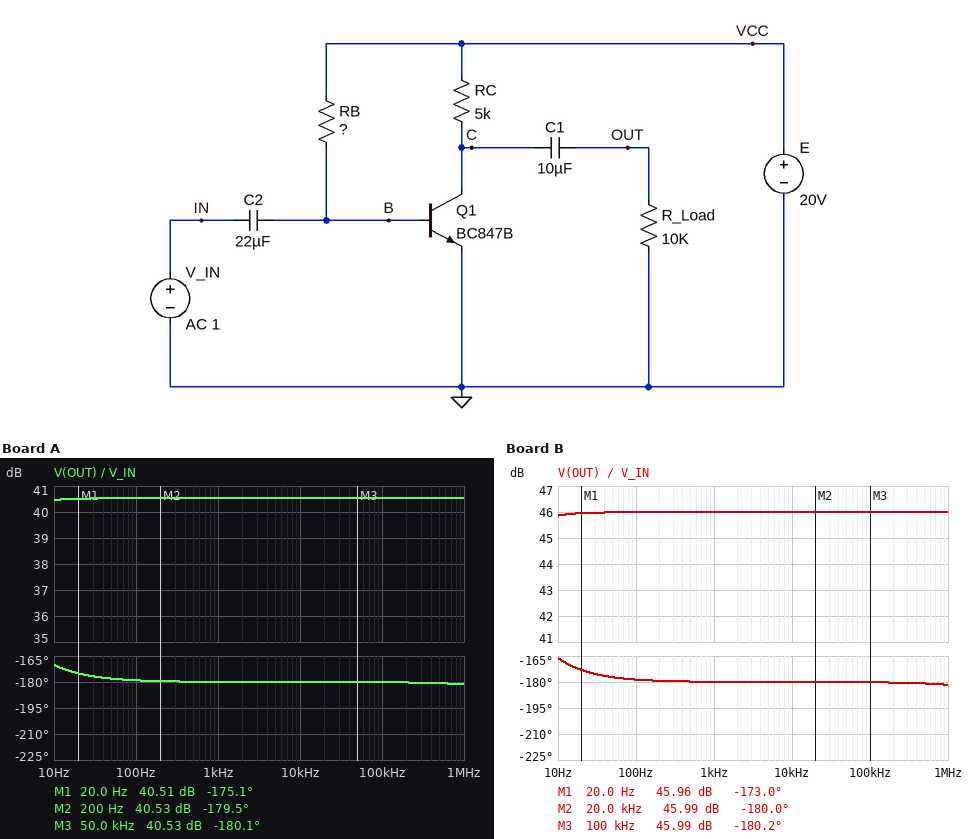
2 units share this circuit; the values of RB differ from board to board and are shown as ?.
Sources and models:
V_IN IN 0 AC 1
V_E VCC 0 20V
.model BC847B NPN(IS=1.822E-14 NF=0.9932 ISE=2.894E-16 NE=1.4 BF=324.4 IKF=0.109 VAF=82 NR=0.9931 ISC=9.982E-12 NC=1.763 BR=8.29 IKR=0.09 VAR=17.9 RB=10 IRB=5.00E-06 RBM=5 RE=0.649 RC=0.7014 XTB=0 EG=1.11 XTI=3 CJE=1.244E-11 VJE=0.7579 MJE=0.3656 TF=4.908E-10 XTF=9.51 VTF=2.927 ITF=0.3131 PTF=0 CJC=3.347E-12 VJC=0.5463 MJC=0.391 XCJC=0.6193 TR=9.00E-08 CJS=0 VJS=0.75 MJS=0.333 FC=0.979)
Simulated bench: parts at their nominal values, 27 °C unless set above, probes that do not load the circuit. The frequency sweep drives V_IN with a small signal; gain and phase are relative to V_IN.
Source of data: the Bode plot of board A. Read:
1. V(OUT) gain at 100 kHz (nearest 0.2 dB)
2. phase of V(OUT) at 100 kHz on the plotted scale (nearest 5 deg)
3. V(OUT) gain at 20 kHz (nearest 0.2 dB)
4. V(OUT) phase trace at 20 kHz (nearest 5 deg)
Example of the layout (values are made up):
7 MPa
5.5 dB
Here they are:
40.6 dB
-180 deg
40.6 dB
-180 deg
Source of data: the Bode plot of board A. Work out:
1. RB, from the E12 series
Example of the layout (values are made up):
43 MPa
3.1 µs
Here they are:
8.2 MΩ
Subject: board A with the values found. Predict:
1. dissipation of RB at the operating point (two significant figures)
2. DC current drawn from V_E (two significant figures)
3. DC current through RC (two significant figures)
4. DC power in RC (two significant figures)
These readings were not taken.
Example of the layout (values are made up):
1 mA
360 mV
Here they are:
46 µW
870 µA
870 µA
3.8 mW
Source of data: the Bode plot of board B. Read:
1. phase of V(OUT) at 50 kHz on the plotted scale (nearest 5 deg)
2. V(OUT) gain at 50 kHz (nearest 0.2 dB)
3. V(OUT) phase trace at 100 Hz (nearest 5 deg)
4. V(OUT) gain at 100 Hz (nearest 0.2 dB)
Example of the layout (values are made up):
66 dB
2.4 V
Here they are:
-180 deg
46.0 dB
-180 deg
46.0 dB
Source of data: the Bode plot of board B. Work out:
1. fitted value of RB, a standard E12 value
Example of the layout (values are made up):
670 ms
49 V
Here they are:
3.9 MΩ
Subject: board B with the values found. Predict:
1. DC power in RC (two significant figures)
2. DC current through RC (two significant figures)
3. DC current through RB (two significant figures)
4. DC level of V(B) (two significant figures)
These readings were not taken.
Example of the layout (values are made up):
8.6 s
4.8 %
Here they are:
15 mW
1.7 mA
5.0 µA
650 mV
